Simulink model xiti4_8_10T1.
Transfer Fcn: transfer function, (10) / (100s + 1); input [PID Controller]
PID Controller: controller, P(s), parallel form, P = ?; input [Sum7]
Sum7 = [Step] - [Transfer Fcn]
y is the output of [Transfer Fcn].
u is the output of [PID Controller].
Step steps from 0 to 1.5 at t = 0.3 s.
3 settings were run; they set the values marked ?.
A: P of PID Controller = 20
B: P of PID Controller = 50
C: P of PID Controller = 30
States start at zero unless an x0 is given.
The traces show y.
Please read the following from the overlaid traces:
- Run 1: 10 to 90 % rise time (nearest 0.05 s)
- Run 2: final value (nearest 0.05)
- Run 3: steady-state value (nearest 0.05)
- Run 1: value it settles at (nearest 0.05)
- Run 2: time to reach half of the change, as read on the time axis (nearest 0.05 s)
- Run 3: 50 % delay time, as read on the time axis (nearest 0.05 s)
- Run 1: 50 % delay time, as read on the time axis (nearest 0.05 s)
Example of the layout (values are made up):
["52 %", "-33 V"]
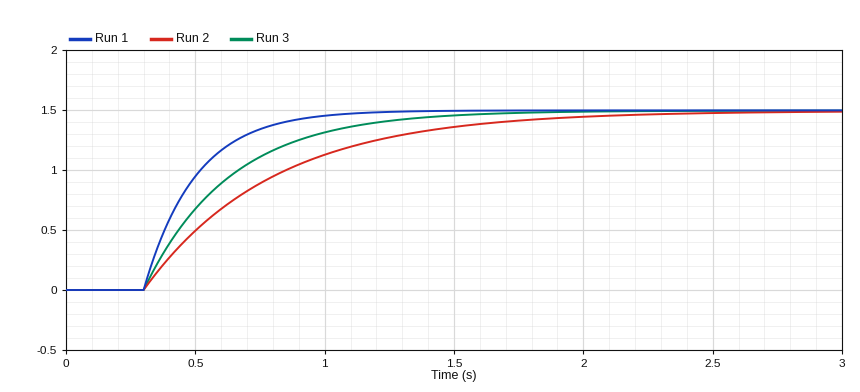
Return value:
["0.45 s", "1.50", "1.50", "1.50", "0.65 s", "0.55 s", "0.45 s"]
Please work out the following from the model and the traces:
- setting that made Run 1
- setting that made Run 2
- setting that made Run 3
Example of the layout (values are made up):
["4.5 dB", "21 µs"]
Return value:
["B", "A", "C"]
